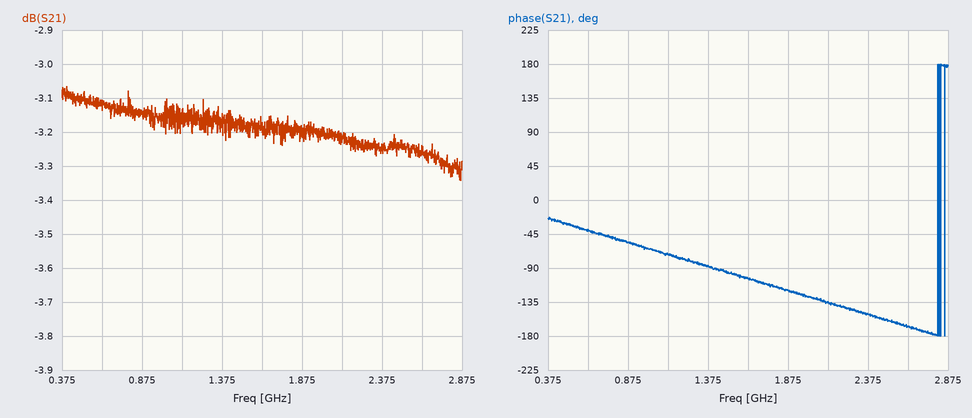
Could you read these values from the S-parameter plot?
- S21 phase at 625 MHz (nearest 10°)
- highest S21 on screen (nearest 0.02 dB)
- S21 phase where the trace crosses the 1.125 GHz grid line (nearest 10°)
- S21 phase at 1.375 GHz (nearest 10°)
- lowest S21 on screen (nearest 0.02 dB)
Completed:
-40°
-3.06 dB
-70°
-90°
-3.34 dB
